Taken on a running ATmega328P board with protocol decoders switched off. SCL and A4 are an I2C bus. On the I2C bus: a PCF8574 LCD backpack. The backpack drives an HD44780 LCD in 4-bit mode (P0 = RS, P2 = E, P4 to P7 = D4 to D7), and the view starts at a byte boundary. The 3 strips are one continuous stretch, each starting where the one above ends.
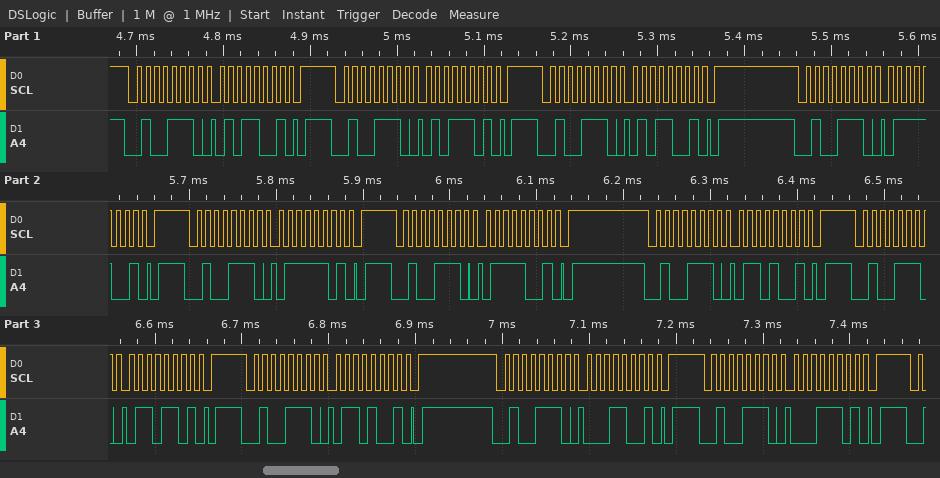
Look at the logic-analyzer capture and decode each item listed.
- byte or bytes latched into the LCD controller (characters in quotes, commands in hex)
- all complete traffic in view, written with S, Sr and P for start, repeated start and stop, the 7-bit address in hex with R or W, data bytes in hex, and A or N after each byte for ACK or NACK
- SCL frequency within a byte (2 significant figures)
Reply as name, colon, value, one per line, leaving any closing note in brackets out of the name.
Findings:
byte or bytes latched into the LCD controller: 'W'
all complete traffic in view, written with S, Sr and P for start, repeated start and stop, the 7-bit address in hex with R or W, data bytes in hex, and A or N after each byte for ACK or NACK: S 27W A 59 A P S 27W A 5D A P S 27W A 59 A P S 27W A 79 A P S 27W A 7D A P S 27W A 79 A P S 27W A 69 A P S 27W A 6D A P S 27W A 69 A P S 27W A 19 A P S 27W A 1D A P
SCL frequency within a byte: 100 kHz
